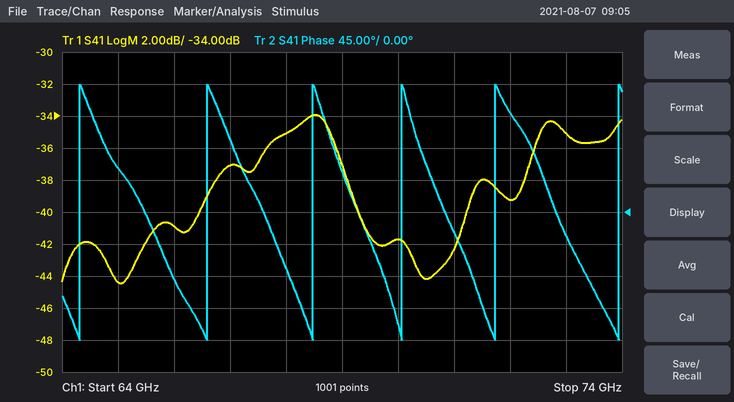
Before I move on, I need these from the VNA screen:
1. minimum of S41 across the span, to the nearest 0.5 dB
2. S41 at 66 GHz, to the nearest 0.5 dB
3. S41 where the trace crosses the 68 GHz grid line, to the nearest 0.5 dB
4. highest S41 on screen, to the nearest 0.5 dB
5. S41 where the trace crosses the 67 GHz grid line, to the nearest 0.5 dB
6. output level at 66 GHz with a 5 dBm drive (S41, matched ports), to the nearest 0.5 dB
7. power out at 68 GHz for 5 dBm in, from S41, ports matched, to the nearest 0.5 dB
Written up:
-44.5 dB
-41.0 dB
-35.0 dB
-34.0 dB
-37.0 dB
-36.0 dBm
-30.0 dBm
